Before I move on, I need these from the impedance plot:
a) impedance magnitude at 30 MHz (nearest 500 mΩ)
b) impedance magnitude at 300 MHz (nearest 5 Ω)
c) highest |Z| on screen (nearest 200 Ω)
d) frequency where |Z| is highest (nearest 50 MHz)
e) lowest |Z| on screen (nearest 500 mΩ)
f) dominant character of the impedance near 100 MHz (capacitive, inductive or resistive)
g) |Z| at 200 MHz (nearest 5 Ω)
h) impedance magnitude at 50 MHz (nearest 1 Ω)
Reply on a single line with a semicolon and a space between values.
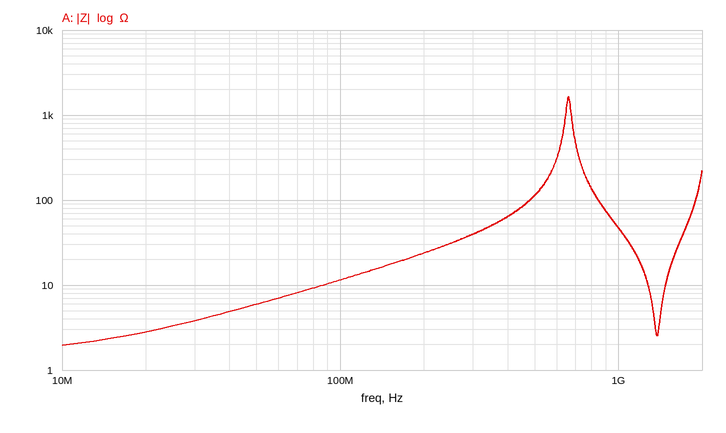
4.0 Ω; 40 Ω; 1.6 kΩ; 650 MHz; 2.0 Ω; inductive; 25 Ω; 6 Ω
